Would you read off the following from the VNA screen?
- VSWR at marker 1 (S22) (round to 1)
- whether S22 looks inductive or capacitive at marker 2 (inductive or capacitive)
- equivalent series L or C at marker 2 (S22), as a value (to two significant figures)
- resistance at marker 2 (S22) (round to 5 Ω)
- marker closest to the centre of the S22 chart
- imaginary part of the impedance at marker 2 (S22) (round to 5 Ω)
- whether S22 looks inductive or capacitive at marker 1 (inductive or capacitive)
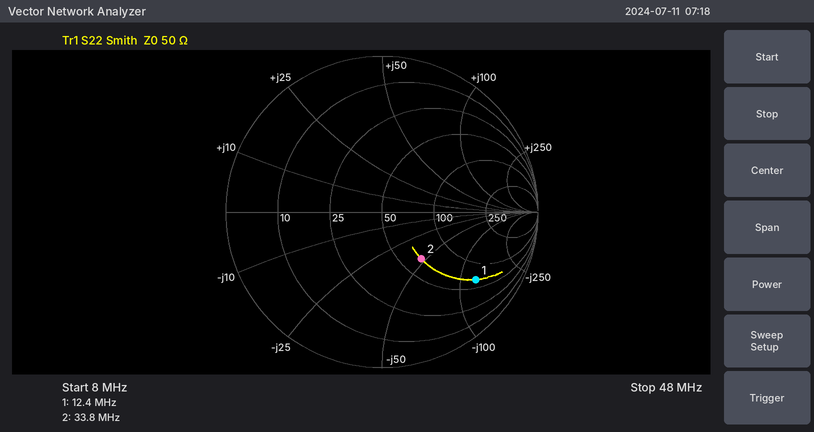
7
capacitive
100 pF
65 Ω
marker 2
-45 Ω
capacitive
